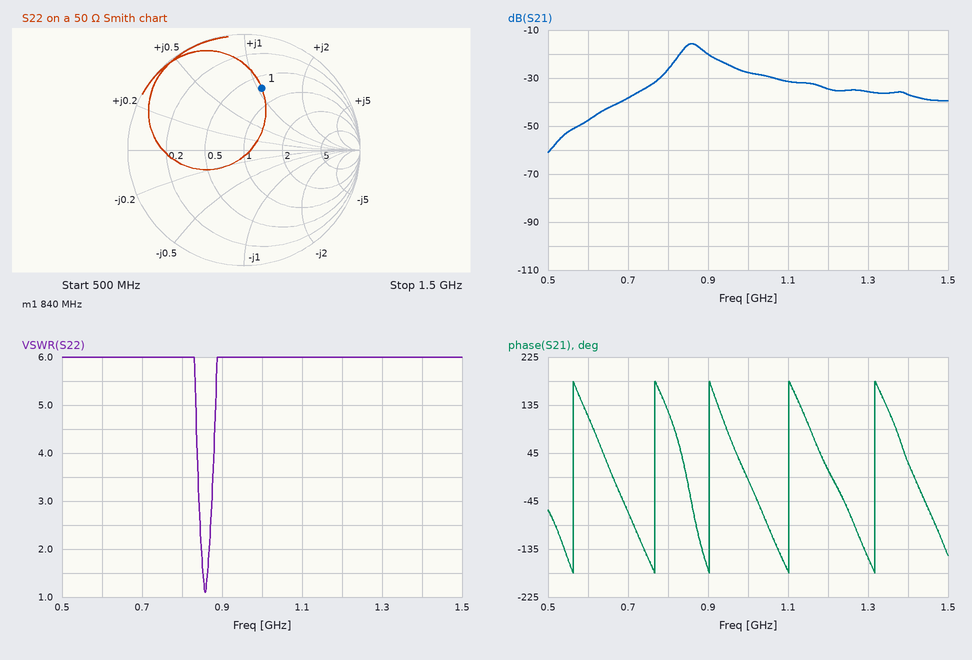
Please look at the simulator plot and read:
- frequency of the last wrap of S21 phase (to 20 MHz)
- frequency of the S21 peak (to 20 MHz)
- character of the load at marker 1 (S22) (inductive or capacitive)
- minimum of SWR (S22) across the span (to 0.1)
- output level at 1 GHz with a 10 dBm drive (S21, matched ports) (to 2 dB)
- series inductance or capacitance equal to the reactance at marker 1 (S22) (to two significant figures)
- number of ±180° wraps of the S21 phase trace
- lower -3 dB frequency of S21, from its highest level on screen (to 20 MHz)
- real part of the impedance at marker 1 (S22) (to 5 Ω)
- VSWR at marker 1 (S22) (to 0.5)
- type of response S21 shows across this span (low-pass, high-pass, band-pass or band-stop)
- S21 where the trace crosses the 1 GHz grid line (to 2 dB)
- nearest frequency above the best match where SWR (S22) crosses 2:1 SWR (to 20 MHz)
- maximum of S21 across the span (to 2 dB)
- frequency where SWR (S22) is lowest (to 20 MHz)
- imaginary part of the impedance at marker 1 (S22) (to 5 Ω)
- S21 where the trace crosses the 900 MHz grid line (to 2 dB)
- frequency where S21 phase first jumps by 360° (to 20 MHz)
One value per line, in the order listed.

1.32 GHz
860 MHz
inductive
1.1
-18 dBm
10 nH
5
840 MHz
35 Ω
3.5
band-pass
-28 dB
860 MHz
-16 dB
860 MHz
+55 Ω
-20 dB
560 MHz
